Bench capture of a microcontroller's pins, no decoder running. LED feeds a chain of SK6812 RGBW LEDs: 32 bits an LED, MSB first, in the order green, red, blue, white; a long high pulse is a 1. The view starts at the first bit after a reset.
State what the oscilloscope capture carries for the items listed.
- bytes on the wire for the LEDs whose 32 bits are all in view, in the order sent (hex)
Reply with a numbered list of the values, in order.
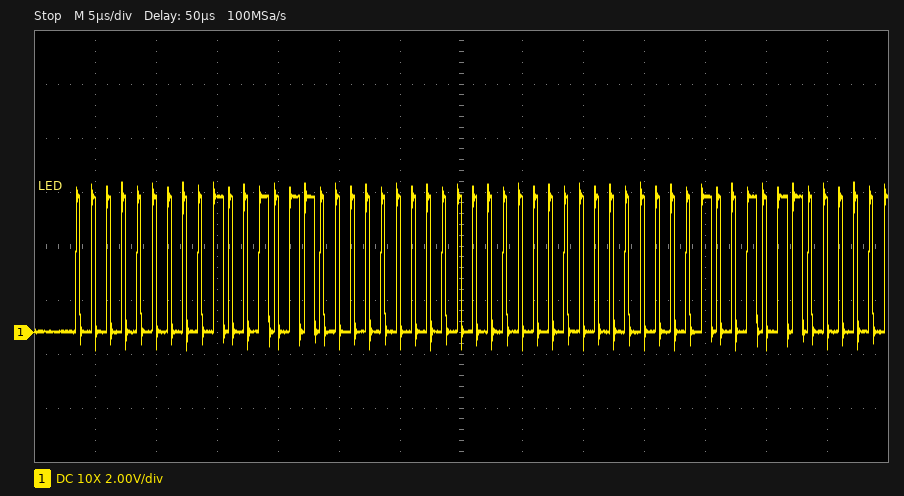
1. 00 4B 00 00
